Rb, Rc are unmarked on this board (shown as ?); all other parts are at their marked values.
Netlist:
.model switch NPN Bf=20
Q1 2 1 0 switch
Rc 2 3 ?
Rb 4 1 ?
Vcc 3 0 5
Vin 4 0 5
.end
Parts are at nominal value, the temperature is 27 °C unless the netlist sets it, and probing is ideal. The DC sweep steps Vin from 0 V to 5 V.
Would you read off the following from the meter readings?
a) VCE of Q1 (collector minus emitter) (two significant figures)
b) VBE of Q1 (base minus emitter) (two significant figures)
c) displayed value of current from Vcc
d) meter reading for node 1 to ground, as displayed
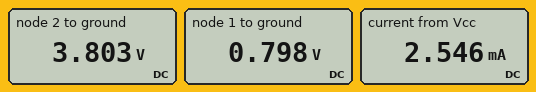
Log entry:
3.8 V
800 mV
2.546 mA
0.798 V
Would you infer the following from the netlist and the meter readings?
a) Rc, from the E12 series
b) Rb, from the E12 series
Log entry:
470 Ω
33 kΩ
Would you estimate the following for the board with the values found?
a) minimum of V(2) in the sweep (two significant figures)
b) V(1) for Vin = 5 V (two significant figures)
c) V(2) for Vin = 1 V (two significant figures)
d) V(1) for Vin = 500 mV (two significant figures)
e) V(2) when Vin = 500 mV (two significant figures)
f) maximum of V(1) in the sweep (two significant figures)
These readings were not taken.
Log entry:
3.8 V
800 mV
4.9 V
500 mV
5.0 V
800 mV
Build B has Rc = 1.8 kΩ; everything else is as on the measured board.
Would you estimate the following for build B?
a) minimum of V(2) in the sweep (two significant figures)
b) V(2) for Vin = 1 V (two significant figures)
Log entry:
420 mV
4.7 V
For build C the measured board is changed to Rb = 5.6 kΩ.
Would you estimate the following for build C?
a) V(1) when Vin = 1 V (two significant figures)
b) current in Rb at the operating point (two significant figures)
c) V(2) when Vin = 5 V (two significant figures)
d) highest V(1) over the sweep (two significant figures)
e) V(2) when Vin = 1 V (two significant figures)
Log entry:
770 mV
740 µA
100 mV
840 mV
4.6 V
